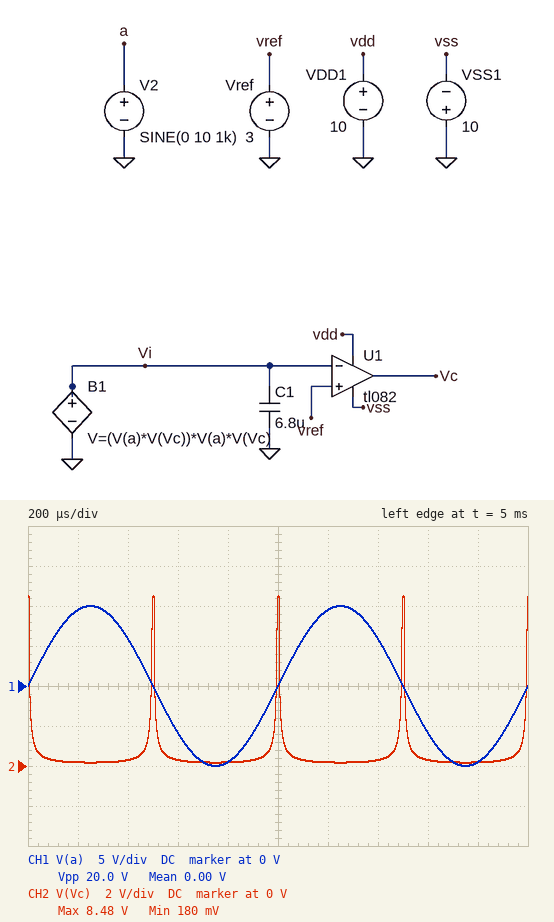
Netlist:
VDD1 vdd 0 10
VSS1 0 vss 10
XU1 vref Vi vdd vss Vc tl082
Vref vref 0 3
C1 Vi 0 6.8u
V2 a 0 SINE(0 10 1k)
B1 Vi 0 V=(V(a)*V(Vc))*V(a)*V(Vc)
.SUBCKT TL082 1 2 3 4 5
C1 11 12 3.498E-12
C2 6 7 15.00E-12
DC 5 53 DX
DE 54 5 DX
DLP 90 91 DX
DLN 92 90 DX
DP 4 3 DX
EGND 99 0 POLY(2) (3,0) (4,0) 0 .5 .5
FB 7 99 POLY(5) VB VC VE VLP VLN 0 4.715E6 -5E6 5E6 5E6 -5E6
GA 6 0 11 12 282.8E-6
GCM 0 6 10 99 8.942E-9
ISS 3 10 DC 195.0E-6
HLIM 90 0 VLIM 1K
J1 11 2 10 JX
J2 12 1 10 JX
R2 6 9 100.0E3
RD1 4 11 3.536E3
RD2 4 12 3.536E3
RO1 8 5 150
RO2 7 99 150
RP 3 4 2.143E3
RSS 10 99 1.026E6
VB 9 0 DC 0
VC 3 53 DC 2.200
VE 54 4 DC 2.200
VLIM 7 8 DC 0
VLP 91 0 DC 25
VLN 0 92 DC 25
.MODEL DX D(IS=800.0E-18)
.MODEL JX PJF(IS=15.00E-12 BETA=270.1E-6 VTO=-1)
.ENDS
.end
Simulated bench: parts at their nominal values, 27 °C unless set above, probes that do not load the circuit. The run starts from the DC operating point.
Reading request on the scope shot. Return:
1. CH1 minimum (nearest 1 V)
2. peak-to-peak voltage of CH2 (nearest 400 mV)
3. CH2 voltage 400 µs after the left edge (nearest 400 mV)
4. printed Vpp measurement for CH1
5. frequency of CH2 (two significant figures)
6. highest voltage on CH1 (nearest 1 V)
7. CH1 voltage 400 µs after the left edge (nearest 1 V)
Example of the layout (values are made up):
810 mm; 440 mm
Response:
-10 V; 8.4 V; 400 mV; 20.0 V; 2.0 kHz; 10 V; 6 V
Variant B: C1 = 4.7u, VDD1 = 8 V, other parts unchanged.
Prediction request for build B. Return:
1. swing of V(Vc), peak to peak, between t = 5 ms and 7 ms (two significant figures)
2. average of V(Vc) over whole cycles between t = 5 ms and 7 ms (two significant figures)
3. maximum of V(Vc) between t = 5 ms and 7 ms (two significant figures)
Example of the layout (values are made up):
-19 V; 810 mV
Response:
6.3 V; 590 mV; 6.5 V
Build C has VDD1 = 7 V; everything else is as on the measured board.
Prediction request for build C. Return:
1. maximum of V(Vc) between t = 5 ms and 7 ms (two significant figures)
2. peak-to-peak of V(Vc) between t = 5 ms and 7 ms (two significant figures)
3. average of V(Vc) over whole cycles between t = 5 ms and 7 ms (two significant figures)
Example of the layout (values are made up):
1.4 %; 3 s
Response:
5.5 V; 5.3 V; 570 mV
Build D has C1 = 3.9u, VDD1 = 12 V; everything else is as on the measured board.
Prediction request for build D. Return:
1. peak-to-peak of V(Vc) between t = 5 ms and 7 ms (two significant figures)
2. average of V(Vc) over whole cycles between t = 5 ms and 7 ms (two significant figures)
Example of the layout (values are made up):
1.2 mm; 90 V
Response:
10 V; 640 mV
